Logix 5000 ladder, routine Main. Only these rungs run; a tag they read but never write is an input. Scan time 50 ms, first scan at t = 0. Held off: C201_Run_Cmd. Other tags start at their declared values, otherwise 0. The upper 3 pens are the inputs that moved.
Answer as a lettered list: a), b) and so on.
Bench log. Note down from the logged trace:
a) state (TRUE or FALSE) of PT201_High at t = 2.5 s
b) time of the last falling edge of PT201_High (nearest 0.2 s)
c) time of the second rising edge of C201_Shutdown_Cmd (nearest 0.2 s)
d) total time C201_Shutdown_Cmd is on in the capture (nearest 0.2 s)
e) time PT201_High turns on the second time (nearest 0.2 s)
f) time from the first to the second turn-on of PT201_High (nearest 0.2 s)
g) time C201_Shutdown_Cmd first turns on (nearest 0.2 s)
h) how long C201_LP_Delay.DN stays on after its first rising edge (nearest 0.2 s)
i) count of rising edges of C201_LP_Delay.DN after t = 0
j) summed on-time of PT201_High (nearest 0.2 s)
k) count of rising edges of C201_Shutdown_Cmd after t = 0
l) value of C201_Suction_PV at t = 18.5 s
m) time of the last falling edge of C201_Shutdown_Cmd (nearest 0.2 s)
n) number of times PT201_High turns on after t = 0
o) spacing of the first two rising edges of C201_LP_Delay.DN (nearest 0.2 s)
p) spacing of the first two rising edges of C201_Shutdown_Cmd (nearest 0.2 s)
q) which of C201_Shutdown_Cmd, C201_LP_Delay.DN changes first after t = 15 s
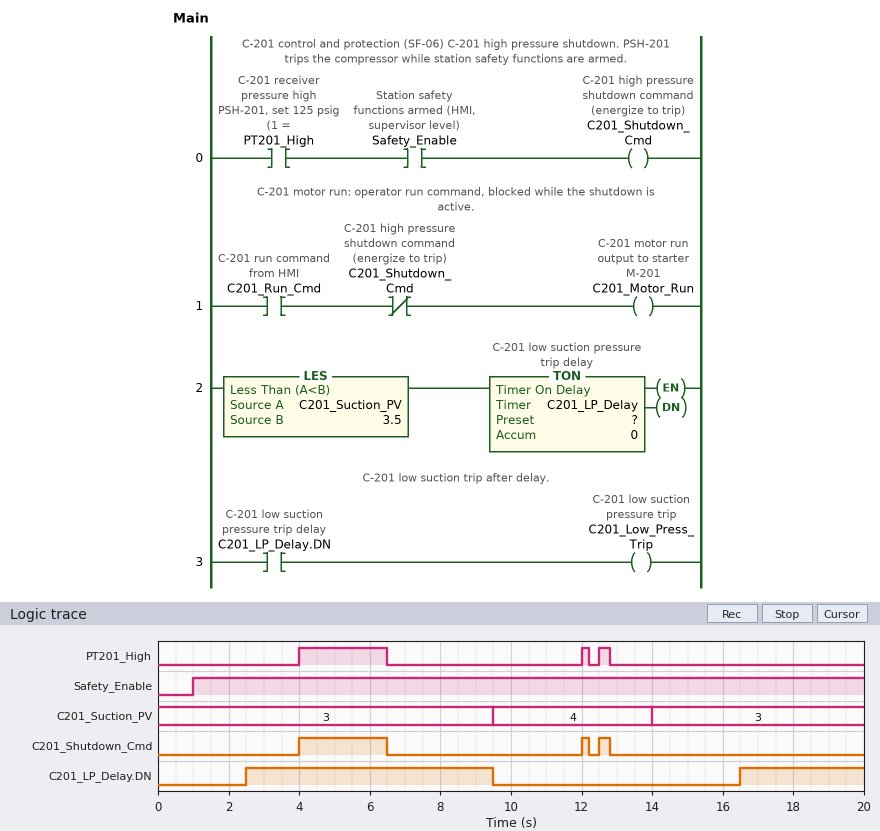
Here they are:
a) FALSE
b) 12.8 s
c) 12.0 s
d) 3.0 s
e) 12.0 s
f) 8.0 s
g) 4.0 s
h) 7.0 s
i) 2
j) 3.0 s
k) 3
l) 3
m) 12.8 s
n) 3
o) 14.0 s
p) 8.0 s
q) C201_LP_Delay.DN
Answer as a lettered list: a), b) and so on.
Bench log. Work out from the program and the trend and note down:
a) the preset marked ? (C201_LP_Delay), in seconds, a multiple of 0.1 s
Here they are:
a) 2.5 s
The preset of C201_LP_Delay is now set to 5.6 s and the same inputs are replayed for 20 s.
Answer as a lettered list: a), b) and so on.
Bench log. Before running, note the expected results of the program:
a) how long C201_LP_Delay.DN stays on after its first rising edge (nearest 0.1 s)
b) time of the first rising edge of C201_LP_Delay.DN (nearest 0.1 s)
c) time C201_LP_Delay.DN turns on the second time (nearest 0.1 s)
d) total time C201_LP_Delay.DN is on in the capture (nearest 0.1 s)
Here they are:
a) 3.9 s
b) 5.6 s
c) 19.6 s
d) 4.3 s
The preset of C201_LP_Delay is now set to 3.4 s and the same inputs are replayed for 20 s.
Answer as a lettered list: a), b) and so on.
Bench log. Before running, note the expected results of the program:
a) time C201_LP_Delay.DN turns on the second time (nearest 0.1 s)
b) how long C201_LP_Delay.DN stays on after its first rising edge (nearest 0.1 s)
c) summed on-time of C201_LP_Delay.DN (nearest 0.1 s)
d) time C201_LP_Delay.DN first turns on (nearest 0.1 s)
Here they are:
a) 17.4 s
b) 6.1 s
c) 8.7 s
d) 3.4 s
